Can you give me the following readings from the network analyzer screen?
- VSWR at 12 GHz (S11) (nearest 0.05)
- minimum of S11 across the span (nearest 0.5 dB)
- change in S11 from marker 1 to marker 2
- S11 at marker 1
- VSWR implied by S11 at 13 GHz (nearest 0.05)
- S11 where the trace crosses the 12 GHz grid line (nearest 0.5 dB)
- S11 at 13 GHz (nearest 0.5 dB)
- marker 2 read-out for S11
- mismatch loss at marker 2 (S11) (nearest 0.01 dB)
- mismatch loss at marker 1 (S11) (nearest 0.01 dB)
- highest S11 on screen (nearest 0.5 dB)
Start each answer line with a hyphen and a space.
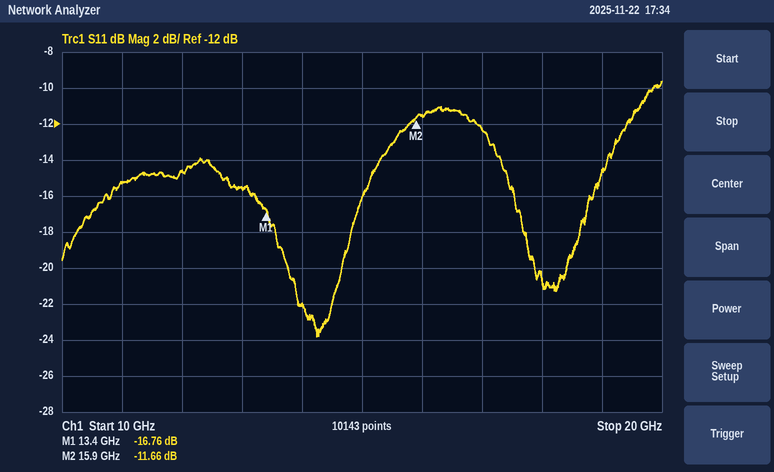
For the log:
- 1.45
- -24.0 dB
- 5.10 dB
- -16.76 dB
- 1.40
- -14.5 dB
- -15.5 dB
- -11.66 dB
- 0.31 dB
- 0.09 dB
- -9.5 dB
